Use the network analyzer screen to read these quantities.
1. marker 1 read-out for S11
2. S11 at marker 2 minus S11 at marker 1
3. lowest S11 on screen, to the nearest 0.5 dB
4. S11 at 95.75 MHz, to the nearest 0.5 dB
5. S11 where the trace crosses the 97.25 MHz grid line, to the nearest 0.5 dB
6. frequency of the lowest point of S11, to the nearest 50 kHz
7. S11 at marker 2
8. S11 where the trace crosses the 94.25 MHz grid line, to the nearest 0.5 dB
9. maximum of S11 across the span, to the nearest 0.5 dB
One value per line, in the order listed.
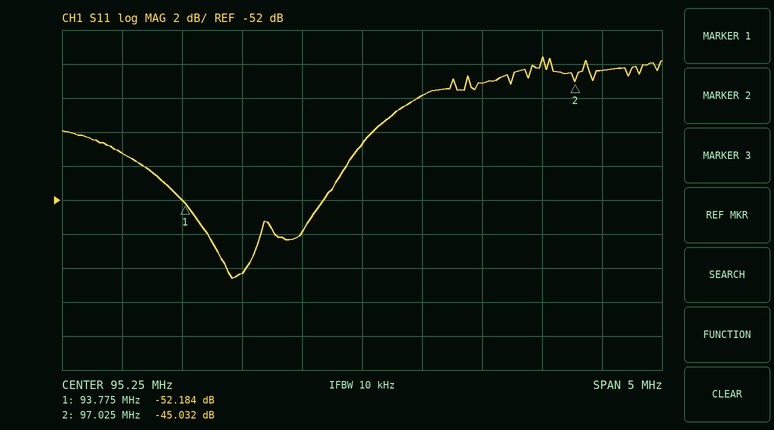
-52.184 dB
7.152 dB
-56.5 dB
-46.0 dB
-44.5 dB
94.15 MHz
-45.032 dB
-56.5 dB
-43.5 dB
